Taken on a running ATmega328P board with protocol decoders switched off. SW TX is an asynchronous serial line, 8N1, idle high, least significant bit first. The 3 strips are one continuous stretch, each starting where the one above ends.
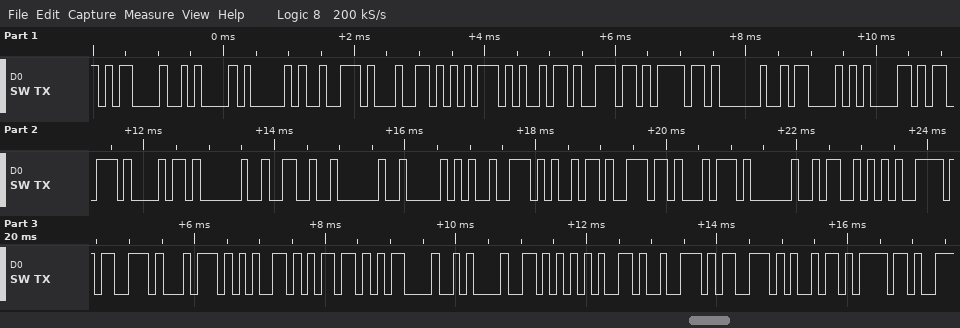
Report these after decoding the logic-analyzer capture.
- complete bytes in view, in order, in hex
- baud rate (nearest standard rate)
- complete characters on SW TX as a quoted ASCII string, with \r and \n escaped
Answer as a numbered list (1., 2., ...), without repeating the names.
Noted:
1. 0D 0A 41 72 64 75 69 6E 6F 20 43 61 73 68 20 26 20 50 72 69 6E 74 20 53 79 73 74 65 6D 0D 0A 56 65 72 73 69 6F
2. 9600 baud
3. "\r\nArduino Cash & Print System\r\nVersio"
